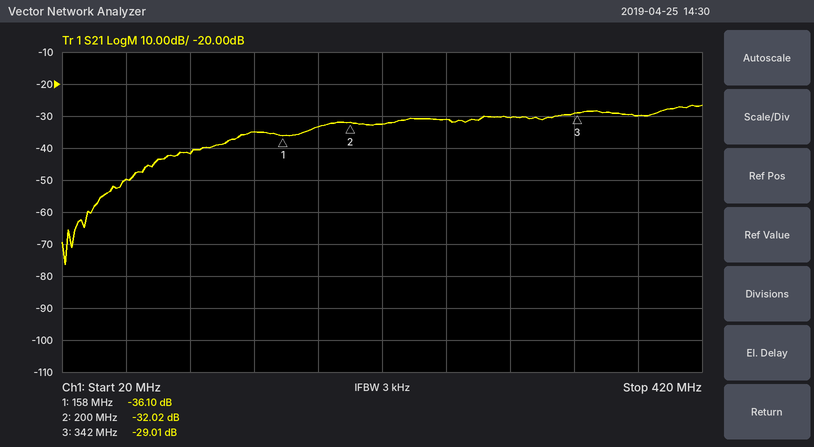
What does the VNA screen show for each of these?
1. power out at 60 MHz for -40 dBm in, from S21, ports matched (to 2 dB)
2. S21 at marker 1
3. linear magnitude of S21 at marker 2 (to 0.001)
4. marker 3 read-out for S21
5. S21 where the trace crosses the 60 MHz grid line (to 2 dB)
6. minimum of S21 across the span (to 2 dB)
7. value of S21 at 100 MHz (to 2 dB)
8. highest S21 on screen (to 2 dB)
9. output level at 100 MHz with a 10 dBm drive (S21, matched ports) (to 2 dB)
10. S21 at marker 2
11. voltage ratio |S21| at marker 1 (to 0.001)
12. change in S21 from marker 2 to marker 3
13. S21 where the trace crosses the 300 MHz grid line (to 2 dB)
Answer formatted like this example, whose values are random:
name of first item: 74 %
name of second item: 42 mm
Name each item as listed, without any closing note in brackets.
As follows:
power out at 60 MHz for -40 dBm in, from S21, ports matched: -90 dBm
S21 at marker 1: -36.10 dB
linear magnitude of S21 at marker 2: 0.025
marker 3 read-out for S21: -29.01 dB
S21 where the trace crosses the 60 MHz grid line: -50 dB
minimum of S21 across the span: -76 dB
value of S21 at 100 MHz: -42 dB
highest S21 on screen: -26 dB
output level at 100 MHz with a 10 dBm drive (S21, matched ports): -32 dBm
S21 at marker 2: -32.02 dB
voltage ratio |S21| at marker 1: 0.016
change in S21 from marker 2 to marker 3: 3.01 dB
S21 where the trace crosses the 300 MHz grid line: -30 dB
